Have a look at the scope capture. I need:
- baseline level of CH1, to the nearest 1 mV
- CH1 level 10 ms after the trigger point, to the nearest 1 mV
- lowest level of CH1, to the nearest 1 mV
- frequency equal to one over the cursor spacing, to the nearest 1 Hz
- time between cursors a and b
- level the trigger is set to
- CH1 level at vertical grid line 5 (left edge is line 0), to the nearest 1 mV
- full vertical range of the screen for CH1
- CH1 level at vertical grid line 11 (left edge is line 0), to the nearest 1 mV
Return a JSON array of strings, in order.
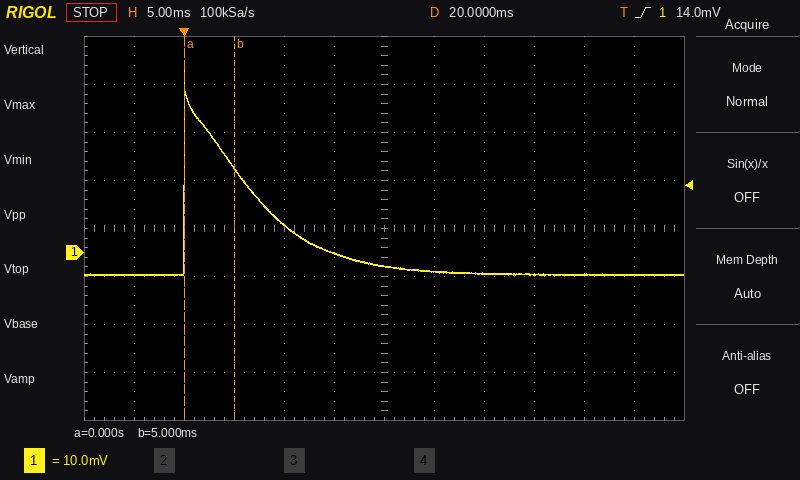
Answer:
["-5 mV", "6 mV", "-5 mV", "200 Hz", "5.0 ms", "14.0 mV", "0 mV", "80 mV", "-5 mV"]
